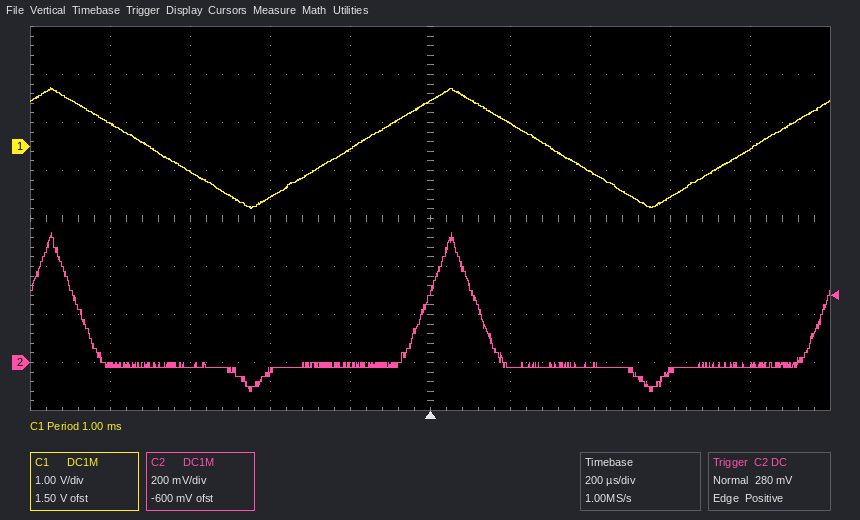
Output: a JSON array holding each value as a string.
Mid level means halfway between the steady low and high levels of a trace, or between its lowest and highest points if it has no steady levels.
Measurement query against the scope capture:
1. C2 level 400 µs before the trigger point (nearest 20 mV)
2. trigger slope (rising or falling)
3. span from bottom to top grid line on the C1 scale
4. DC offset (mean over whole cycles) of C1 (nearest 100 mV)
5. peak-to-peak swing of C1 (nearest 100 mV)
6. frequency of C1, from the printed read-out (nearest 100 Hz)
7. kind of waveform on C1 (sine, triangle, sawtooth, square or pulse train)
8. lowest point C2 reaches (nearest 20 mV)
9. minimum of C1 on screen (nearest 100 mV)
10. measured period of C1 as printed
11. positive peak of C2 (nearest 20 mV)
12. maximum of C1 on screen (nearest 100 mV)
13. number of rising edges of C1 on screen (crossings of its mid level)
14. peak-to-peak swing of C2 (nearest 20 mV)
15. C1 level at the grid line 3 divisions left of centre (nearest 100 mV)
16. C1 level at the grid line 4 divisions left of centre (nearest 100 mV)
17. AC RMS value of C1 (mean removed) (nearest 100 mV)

["-40 mV", "rising", "8 V", "0.0 V", "2.5 V", "1.0 kHz", "triangle", "-120 mV", "-1.3 V", "1.00 ms", "540 mV", "1.2 V", "2", "660 mV", "-500 mV", "500 mV", "700 mV"]
